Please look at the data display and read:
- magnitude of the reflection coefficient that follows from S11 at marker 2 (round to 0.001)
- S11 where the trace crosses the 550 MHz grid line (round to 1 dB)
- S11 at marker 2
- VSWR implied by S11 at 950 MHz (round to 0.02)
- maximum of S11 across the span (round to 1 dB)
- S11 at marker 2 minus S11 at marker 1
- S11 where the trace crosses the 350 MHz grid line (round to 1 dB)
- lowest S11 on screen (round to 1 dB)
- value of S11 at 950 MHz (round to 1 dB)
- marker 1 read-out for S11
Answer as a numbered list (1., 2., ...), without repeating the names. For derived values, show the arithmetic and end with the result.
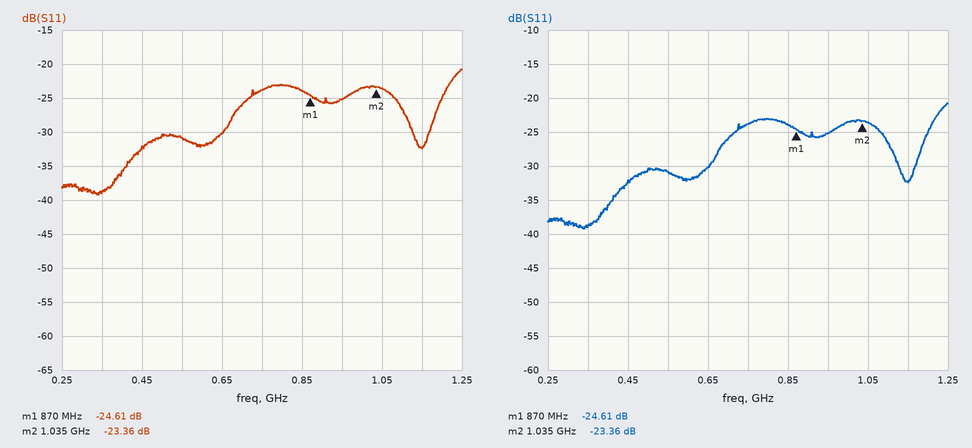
1. 10^(-23.36/20) ≈ 0.068
2. -31 dB
3. -23.36 dB
4. |Γ| = 10^(-25/20) = 0.0562; VSWR = (1 + 0.0562)/(1 − 0.0562) ≈ 1.12
5. -21 dB
6. -23.36 − (-24.61) = 1.25 dB
7. -39 dB
8. -39 dB
9. -25 dB
10. -24.61 dB
